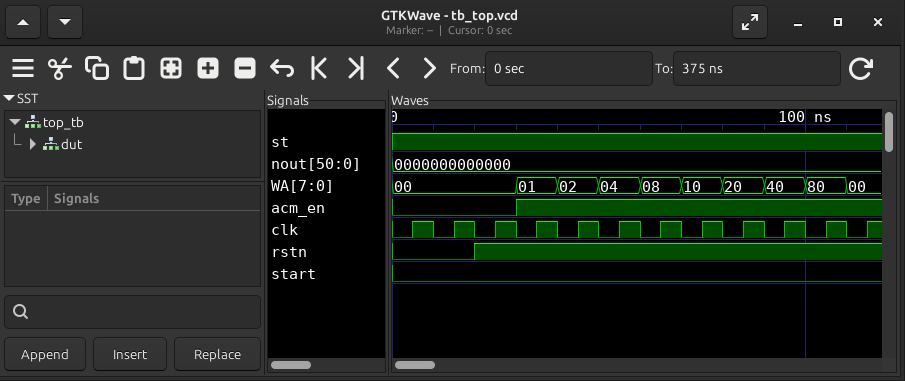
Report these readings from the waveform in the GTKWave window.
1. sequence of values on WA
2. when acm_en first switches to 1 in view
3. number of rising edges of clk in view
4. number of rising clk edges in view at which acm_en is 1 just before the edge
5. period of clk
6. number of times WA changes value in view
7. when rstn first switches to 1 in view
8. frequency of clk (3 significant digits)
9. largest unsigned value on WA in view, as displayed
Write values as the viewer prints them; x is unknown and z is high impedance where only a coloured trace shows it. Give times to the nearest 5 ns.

00, 01, 02, 04, 08, 10, 20, 40, 80, 00
30 ns
12
9
10 ns
9
20 ns
100 MHz
80
